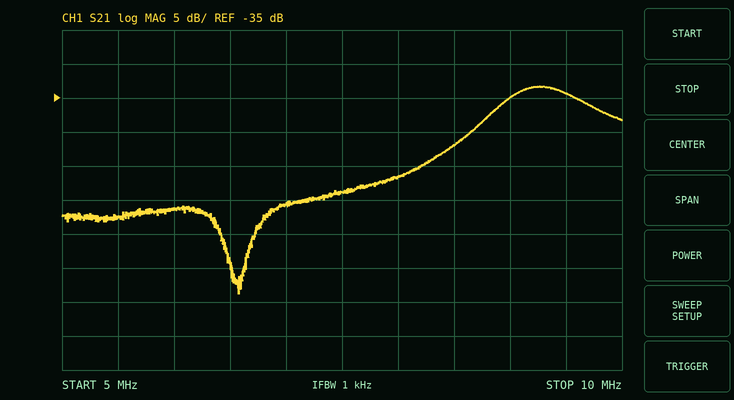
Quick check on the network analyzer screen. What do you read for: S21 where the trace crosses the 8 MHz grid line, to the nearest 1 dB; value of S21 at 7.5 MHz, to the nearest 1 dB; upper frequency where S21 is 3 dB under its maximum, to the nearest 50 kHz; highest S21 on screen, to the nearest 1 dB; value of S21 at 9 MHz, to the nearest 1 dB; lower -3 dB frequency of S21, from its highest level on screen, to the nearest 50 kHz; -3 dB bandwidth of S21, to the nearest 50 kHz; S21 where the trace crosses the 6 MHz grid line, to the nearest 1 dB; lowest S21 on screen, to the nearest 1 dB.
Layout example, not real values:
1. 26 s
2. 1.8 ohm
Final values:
1. -47 dB
2. -49 dB
3. 9.75 MHz
4. -33 dB
5. -35 dB
6. 8.90 MHz
7. 850 kHz
8. -51 dB
9. -64 dB
